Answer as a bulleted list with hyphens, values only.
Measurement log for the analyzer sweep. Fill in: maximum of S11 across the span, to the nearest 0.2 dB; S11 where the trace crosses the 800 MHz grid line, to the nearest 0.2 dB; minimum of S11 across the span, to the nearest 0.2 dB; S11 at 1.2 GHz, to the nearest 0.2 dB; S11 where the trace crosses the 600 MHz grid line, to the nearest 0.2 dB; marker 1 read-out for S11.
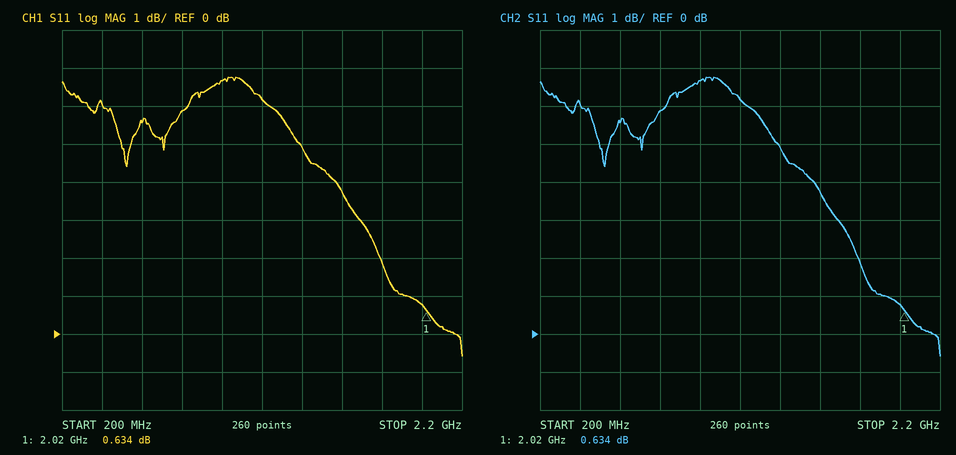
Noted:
- 6.8 dB
- 5.8 dB
- -0.6 dB
- 6.2 dB
- 5.6 dB
- 0.634 dB
